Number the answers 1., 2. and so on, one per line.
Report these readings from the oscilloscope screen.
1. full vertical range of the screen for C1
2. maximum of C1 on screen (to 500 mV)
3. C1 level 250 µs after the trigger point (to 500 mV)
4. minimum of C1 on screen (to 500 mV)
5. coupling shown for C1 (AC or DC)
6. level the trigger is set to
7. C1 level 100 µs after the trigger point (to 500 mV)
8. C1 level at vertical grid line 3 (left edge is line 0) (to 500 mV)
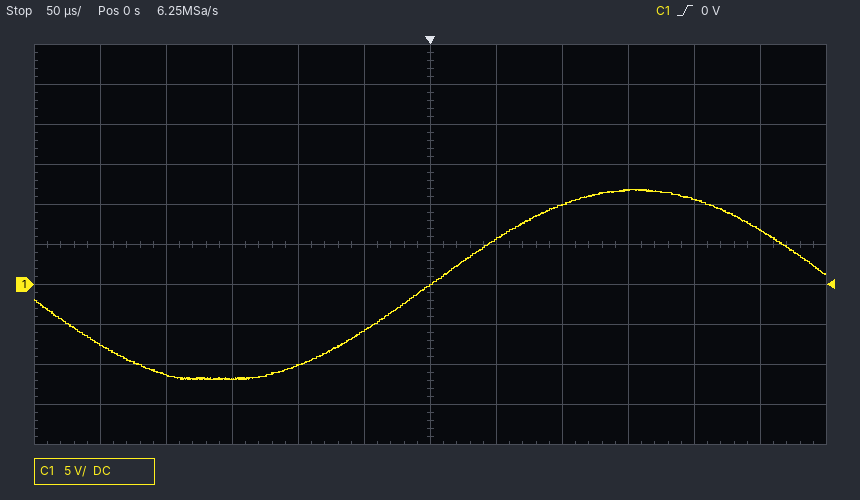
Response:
1. 50 V
2. 12.0 V
3. 7.0 V
4. -12.0 V
5. DC
6. 0 V
7. 10.0 V
8. -12.0 V
